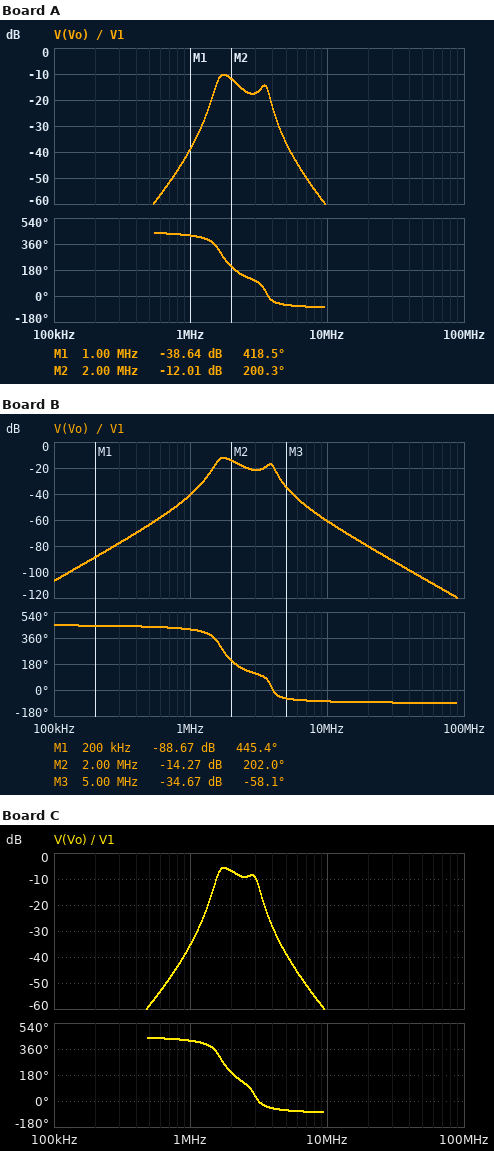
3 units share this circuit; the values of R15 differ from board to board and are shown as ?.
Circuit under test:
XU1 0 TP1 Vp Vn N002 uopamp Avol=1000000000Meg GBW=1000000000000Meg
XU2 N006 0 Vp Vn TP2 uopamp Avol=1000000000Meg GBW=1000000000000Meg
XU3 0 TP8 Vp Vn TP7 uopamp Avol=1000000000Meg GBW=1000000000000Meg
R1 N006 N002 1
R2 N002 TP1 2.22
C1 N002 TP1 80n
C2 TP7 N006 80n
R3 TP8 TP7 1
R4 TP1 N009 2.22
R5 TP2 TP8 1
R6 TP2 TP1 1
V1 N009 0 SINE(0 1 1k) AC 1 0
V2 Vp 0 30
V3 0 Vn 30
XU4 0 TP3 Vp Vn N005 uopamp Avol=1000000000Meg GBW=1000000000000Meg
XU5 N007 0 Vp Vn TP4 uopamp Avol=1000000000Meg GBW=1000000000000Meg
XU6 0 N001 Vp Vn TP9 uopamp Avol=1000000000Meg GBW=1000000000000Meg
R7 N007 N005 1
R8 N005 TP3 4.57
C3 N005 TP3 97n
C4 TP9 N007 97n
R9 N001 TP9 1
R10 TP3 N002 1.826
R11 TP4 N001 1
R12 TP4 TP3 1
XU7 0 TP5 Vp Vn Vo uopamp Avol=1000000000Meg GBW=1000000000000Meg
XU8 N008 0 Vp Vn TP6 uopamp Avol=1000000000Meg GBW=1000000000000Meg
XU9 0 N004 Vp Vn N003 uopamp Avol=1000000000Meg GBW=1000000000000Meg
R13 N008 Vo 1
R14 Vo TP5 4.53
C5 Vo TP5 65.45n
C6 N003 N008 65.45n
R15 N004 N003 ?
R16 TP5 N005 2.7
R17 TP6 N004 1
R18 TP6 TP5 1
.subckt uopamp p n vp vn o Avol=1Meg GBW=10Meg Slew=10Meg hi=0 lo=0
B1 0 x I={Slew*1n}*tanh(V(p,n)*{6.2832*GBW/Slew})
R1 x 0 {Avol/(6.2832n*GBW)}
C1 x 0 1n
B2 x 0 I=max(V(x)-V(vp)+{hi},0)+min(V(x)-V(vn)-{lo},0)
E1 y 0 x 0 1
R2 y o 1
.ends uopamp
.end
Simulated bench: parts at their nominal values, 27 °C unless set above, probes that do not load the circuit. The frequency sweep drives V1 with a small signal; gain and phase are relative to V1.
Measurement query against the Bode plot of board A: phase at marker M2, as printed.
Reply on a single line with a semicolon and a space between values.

200.3 deg
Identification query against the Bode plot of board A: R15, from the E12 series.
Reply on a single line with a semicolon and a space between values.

0.47 Ω
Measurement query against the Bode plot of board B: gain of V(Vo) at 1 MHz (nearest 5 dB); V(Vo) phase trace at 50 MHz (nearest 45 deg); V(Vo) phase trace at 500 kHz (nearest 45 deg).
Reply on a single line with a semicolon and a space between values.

-40 dB; -90 deg; 450 deg
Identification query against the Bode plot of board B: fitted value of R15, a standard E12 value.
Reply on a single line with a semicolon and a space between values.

0.39 Ω
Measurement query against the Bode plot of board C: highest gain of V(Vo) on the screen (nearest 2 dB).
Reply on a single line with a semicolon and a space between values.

-6 dB
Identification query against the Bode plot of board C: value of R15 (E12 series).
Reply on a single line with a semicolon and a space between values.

0.68 Ω
